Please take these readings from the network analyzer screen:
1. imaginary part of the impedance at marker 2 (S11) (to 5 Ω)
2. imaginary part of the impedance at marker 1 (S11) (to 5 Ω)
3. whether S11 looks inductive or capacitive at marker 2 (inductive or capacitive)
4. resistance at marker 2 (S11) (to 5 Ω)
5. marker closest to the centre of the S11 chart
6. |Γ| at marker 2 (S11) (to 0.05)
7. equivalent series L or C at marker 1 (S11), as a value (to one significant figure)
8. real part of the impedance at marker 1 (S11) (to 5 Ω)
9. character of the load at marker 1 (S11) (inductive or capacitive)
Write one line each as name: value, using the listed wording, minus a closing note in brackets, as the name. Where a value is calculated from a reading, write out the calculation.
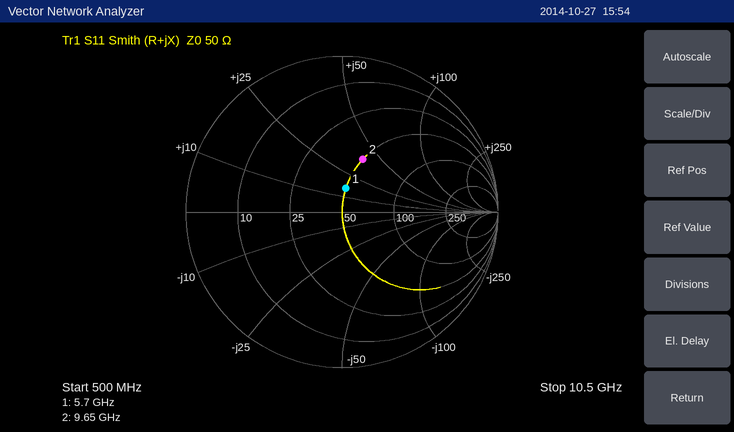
imaginary part of the impedance at marker 2 (S11): +40 Ω
imaginary part of the impedance at marker 1 (S11): +15 Ω
whether S11 looks inductive or capacitive at marker 2: inductive
resistance at marker 2 (S11): 50 Ω
marker closest to the centre of the S11 chart: marker 1
|Γ| at marker 2 (S11): 0.35
equivalent series L or C at marker 1 (S11), as a value: L = 15 Ω/(2π × 5.7 GHz) ≈ 419 pH, so 400 pH to one significant figure
real part of the impedance at marker 1 (S11): 50 Ω
character of the load at marker 1 (S11): inductive
